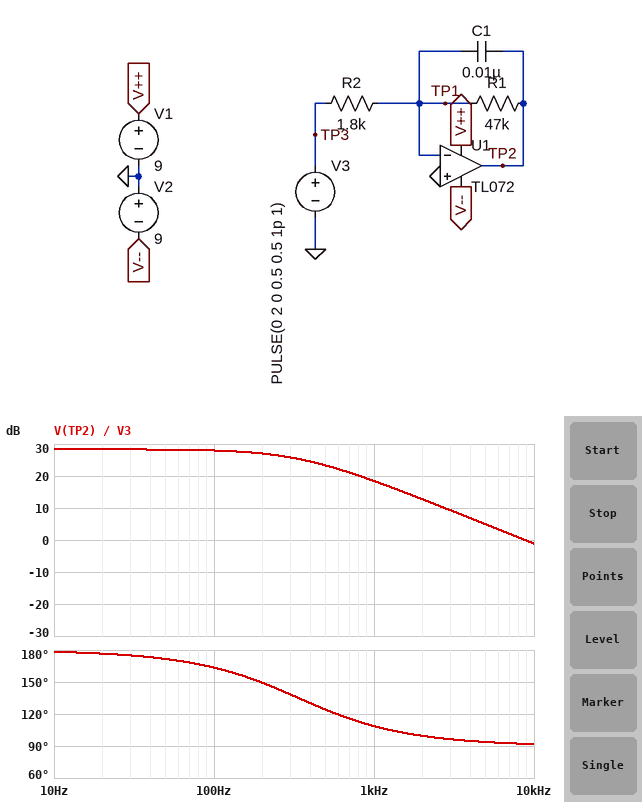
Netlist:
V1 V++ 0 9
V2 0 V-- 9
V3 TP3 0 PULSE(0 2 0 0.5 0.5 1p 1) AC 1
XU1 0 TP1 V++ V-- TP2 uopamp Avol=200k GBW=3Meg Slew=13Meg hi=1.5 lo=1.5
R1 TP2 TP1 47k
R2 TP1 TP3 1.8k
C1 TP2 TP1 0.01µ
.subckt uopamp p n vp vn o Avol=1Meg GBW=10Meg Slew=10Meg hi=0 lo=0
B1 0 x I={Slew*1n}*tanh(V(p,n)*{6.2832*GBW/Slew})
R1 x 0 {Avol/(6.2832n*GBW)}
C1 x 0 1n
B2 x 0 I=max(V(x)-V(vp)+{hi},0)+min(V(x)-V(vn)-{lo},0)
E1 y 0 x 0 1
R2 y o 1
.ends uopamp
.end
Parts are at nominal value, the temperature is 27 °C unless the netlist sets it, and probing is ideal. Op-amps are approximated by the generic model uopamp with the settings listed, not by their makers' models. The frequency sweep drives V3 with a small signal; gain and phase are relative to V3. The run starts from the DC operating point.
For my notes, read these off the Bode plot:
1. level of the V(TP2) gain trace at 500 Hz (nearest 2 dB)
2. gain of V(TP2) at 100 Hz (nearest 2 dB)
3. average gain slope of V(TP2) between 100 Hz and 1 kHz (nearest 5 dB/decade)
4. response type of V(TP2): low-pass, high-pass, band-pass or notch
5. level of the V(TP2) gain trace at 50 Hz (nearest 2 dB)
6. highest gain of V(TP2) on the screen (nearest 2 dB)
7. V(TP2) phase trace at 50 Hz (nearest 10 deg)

24 dB
28 dB
-10 dB/decade
low-pass
28 dB
28 dB
170 deg
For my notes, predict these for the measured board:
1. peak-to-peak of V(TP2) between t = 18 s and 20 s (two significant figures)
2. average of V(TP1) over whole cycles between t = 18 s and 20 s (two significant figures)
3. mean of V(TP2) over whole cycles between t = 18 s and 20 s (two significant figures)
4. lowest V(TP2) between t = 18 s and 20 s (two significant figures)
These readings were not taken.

7.5 V
710 mV
-7.0 V
-7.5 V
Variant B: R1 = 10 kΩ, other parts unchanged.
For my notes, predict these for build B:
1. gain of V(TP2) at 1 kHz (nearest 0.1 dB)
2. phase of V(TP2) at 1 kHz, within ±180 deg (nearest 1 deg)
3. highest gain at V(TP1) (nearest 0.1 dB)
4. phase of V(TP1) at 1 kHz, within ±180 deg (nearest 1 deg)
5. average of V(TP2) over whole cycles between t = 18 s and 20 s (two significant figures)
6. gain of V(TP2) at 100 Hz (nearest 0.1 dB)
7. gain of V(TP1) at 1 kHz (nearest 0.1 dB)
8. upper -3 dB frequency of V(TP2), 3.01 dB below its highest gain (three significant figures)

13.4 dB
148 deg
-50.6 dB
57 deg
-5.0 V
14.9 dB
-56.1 dB
1.59 kHz
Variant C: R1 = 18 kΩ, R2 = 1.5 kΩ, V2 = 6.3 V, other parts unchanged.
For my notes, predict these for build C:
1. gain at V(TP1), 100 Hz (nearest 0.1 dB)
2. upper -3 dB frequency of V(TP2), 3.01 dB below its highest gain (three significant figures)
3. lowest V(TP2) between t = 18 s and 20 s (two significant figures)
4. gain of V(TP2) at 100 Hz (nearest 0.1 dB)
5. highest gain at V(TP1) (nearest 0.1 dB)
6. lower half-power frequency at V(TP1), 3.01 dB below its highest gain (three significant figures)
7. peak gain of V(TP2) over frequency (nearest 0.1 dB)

-67.9 dB
881 Hz
-4.8 V
21.5 dB
-49.1 dB
880 Hz
21.6 dB
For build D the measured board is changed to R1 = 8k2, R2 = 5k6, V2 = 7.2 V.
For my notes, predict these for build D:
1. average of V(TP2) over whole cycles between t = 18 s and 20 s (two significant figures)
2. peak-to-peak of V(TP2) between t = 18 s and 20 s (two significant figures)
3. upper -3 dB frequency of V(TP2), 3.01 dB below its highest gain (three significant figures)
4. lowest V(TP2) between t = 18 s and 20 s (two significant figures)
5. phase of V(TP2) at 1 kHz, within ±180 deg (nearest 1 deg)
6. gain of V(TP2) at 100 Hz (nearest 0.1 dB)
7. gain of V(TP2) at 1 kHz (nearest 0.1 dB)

-1.5 V
2.9 V
1.94 kHz
-2.9 V
153 deg
3.3 dB
2.3 dB
